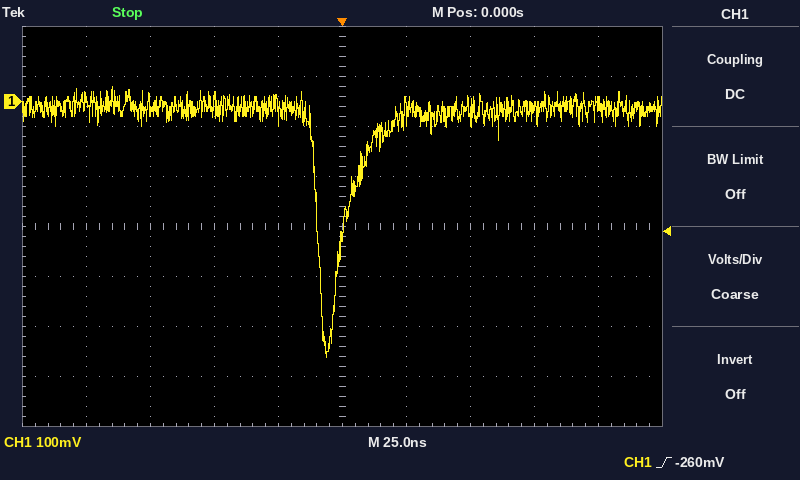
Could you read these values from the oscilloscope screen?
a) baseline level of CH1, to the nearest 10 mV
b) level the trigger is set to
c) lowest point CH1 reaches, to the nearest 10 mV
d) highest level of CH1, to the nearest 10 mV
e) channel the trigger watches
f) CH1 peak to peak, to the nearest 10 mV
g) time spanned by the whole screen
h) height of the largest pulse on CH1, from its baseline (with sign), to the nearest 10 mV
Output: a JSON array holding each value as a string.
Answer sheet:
["-10 mV", "-260 mV", "-510 mV", "30 mV", "CH1", "540 mV", "250 ns", "-500 mV"]
